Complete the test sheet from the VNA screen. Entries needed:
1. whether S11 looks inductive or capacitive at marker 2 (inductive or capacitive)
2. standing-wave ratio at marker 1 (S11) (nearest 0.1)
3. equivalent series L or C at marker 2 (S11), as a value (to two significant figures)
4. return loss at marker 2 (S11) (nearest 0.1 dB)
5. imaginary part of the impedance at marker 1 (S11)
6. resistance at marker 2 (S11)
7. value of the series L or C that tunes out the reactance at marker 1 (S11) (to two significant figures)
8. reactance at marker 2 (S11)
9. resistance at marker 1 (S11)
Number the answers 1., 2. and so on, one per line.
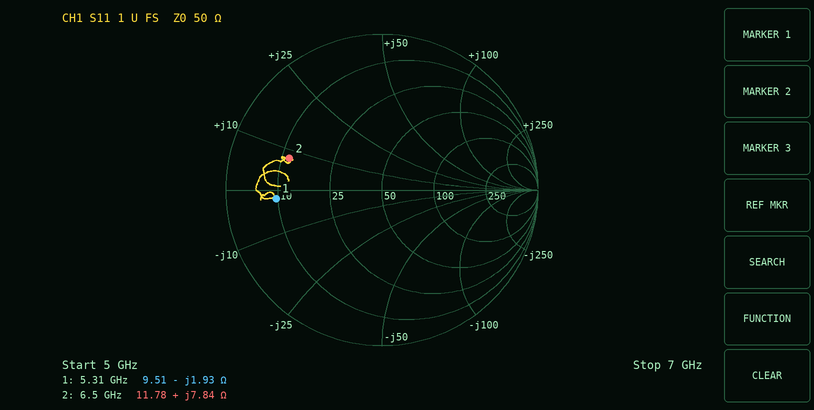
1. inductive
2. 5.3
3. 190 pH
4. 4.1 dB
5. -1.93 Ω
6. 11.78 Ω
7. 58 pH
8. +7.84 Ω
9. 9.51 Ω
